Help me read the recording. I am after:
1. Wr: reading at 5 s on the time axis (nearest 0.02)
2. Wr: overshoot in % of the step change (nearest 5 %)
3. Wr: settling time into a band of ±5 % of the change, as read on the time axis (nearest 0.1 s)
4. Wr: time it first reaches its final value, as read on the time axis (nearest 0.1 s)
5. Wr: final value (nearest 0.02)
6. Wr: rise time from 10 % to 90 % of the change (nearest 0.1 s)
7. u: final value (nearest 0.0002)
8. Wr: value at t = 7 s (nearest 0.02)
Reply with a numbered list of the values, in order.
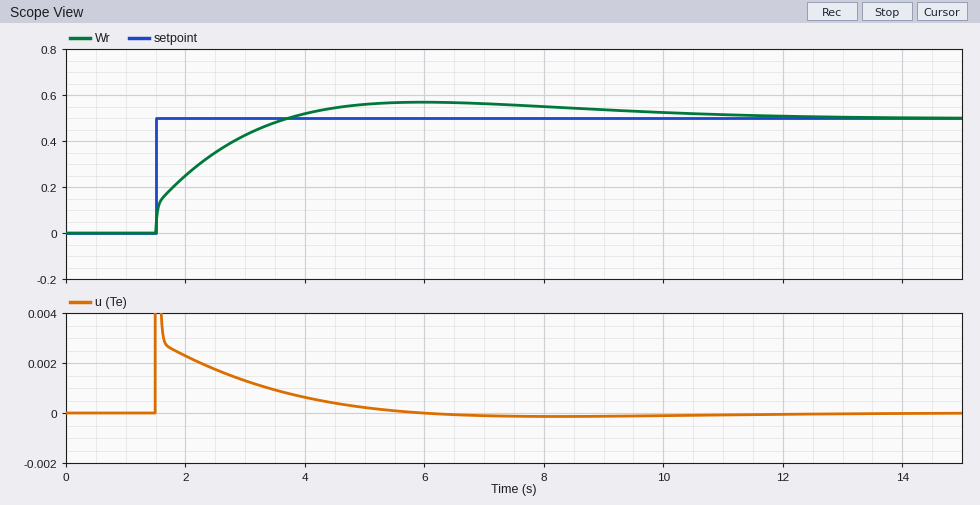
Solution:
1. 0.56
2. 15 %
3. 9.9 s
4. 3.7 s
5. 0.50
6. 1.7 s
7. 0.0000
8. 0.56
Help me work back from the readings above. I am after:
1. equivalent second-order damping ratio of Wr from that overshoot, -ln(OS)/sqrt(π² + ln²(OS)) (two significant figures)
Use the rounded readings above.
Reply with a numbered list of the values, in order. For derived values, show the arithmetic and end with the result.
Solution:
1. ln(0.15) = -1.897; 1.897 / sqrt(9.870 + 3.599) = 0.52
